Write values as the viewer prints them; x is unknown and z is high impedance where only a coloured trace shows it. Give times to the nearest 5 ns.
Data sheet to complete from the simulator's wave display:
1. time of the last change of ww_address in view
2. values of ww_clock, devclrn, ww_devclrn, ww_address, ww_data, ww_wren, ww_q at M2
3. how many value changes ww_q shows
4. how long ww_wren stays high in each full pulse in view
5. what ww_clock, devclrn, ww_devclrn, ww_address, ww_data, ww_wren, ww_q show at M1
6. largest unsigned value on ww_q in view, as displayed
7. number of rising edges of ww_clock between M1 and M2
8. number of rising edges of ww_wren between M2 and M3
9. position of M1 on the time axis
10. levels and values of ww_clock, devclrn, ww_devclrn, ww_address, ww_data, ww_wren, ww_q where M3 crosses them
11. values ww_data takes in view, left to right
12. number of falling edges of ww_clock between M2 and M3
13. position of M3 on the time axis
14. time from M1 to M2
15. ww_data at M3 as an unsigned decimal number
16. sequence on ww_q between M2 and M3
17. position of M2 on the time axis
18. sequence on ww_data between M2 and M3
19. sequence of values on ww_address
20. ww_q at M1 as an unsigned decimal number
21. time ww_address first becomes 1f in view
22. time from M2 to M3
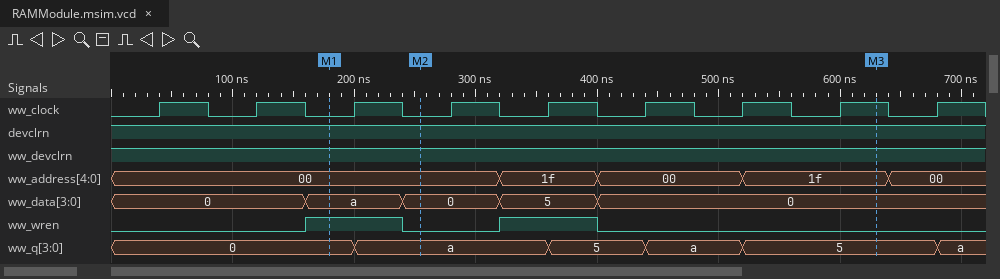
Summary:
640 ns
ww_clock=0, devclrn=1, ww_devclrn=1, ww_address=00, ww_data=0, ww_wren=0, ww_q=a
5
80 ns, 80 ns
ww_clock=0, devclrn=1, ww_devclrn=1, ww_address=00, ww_data=a, ww_wren=1, ww_q=0
a
1
1
180 ns
ww_clock=1, devclrn=1, ww_devclrn=1, ww_address=1f, ww_data=0, ww_wren=0, ww_q=5
0, a, 0, 5, 0
4
630 ns
75 ns
0
a, 5, a, 5
255 ns
0, 5, 0
00, 1f, 00, 1f, 00
0
320 ns
375 ns
